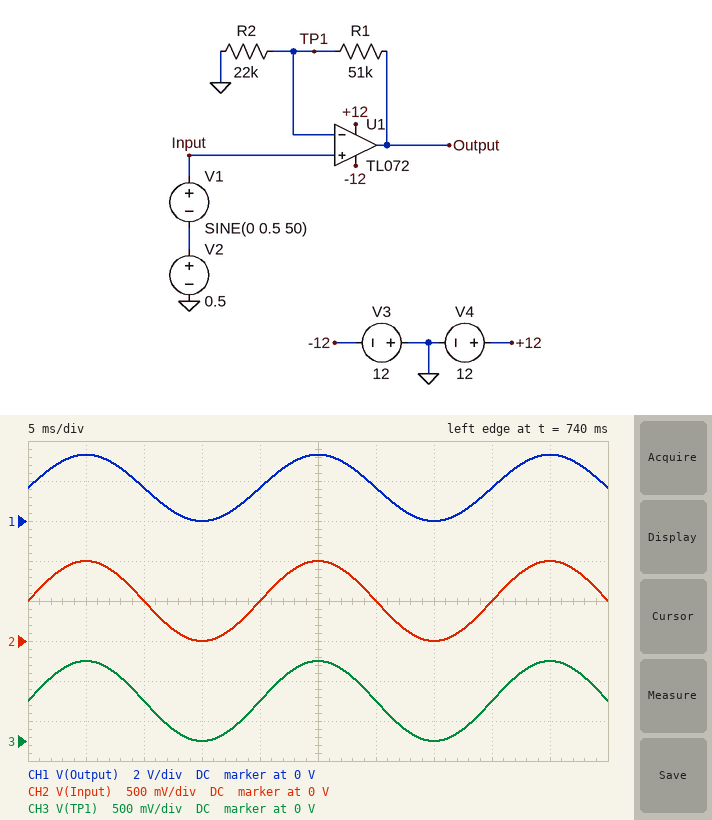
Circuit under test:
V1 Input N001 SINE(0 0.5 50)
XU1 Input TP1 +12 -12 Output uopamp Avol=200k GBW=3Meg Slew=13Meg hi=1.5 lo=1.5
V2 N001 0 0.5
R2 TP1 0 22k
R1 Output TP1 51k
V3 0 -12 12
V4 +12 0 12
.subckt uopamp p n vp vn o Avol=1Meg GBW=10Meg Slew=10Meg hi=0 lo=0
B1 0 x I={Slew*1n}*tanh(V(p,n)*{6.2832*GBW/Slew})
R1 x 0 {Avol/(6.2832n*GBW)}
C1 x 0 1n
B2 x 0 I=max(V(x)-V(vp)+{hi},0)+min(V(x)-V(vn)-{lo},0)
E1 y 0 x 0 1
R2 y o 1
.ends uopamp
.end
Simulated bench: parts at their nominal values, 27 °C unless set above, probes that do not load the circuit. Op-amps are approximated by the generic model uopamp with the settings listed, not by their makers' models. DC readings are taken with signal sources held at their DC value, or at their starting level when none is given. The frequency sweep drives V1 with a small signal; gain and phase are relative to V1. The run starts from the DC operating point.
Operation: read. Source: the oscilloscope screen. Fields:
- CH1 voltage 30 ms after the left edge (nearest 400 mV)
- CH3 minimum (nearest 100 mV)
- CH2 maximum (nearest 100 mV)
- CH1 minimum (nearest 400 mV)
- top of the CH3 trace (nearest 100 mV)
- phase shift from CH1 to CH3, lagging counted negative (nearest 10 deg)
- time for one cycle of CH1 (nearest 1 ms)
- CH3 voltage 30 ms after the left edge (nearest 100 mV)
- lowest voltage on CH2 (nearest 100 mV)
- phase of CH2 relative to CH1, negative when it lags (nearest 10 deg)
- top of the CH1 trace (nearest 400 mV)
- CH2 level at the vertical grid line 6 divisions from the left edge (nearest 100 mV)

1.6 V
0 V
1.0 V
0 V
1.0 V
0 deg
20 ms
500 mV
0 V
0 deg
3.2 V
500 mV
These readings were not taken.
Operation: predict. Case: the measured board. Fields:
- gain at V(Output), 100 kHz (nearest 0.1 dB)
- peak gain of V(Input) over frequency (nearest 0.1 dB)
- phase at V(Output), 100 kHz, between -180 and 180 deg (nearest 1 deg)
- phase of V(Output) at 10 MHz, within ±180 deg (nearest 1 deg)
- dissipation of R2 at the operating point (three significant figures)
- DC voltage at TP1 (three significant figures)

10.4 dB
0 dB
-6 deg
-85 deg
11.4 µW
500 mV
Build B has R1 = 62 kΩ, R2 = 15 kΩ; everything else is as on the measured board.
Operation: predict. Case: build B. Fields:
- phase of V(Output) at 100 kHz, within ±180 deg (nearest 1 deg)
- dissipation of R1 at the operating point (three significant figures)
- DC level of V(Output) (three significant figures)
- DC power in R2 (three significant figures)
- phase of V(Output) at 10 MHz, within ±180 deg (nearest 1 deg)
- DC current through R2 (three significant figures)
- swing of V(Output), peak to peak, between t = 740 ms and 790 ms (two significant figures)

-10 deg
68.9 µW
2.57 V
16.7 µW
-87 deg
33.3 µA
5.1 V
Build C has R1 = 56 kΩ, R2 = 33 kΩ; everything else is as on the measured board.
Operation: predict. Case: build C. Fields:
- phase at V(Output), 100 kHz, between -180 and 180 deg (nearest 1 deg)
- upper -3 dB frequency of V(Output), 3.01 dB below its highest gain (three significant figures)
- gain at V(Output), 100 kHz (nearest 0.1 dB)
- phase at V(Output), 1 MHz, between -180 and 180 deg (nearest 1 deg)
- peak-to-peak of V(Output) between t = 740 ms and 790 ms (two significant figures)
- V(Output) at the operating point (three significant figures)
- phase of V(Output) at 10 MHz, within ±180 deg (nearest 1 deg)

-5 deg
1.11 MHz
8.6 dB
-42 deg
2.7 V
1.35 V
-84 deg
